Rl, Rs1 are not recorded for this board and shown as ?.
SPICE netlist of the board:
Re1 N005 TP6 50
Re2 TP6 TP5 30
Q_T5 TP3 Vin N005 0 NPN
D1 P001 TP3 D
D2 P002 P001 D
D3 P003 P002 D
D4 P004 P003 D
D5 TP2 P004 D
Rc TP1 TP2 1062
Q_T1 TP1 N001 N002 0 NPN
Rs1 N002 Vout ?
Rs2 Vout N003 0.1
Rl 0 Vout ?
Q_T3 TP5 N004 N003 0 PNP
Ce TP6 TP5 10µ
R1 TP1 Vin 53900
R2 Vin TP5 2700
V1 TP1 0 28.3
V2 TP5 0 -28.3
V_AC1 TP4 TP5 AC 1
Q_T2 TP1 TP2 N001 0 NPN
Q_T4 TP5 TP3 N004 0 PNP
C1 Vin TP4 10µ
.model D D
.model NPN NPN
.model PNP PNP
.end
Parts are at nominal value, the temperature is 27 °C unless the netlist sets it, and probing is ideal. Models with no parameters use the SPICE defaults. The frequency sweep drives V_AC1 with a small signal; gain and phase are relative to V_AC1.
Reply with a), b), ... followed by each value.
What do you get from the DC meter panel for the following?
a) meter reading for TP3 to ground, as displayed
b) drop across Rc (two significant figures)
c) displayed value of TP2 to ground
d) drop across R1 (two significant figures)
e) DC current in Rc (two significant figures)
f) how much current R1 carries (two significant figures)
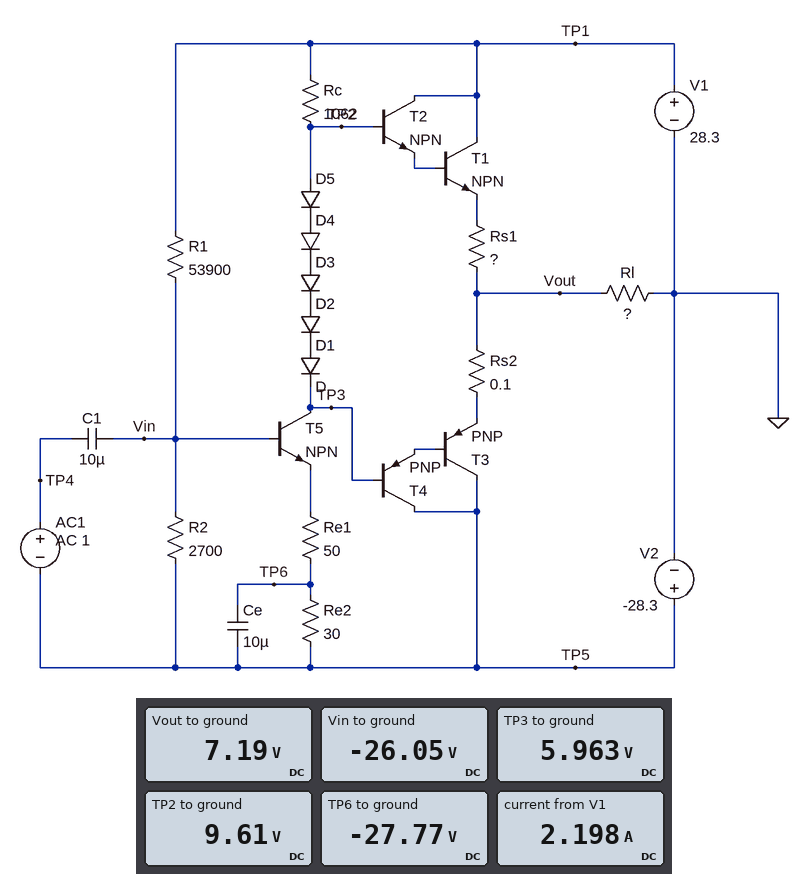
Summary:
a) 5.963 V
b) 19 V
c) 9.61 V
d) 54 V
e) 18 mA
f) 1.0 mA
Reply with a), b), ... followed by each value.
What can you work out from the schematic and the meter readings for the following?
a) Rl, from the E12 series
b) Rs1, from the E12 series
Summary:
a) 3.3 Ω
b) 0.27 Ω
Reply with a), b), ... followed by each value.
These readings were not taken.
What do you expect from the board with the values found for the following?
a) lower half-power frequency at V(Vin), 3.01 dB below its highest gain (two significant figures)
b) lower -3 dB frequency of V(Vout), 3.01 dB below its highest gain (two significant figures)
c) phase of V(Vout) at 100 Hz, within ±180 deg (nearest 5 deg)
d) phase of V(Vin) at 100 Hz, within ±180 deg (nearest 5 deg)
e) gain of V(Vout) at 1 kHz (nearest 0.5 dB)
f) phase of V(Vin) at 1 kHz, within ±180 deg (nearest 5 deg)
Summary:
a) 8.1 Hz
b) 380 Hz
c) -170 deg
d) 5 deg
e) 24.0 dB
f) 0 deg
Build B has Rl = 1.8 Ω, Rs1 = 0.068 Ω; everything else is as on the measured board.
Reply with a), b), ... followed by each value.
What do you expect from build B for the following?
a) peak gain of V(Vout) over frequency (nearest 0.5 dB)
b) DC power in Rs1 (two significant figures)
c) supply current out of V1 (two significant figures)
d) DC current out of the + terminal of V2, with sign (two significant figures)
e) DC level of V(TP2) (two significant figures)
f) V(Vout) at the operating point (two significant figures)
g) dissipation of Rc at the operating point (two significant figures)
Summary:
a) 25.5 dB
b) 1.1 W
c) 4.1 A
d) -23 mA
e) 9.4 V
f) 7.3 V
g) 340 mW
